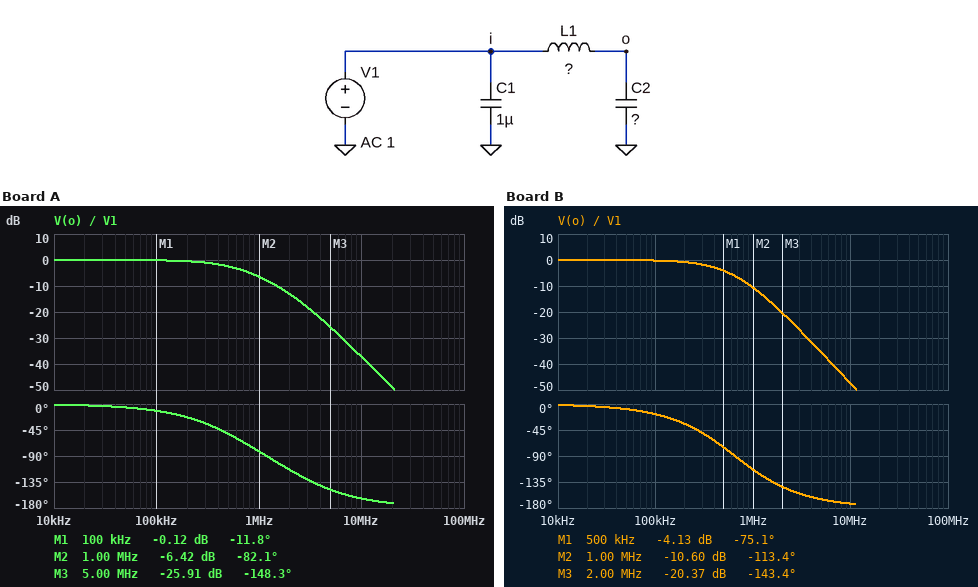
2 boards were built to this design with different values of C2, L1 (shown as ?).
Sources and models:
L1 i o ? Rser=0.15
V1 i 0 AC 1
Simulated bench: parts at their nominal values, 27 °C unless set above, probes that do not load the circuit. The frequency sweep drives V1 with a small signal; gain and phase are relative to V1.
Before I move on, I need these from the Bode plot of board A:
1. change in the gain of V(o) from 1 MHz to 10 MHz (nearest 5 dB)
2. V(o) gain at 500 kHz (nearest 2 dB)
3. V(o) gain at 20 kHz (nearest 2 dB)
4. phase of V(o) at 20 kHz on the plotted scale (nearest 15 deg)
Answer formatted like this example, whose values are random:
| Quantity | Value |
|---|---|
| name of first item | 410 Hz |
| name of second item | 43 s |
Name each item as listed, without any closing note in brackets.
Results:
| Quantity | Value |
|---|---|
| change in the gain of V(o) from 1 MHz to 10 MHz | -30 dB |
| V(o) gain at 500 kHz | -2 dB |
| V(o) gain at 20 kHz | 0 dB |
| phase of V(o) at 20 kHz on the plotted scale | 0 deg |
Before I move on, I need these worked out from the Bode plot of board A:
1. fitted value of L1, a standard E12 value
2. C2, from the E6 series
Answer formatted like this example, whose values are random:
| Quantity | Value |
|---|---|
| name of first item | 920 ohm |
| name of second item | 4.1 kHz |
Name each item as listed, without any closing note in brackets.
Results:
| Quantity | Value |
|---|---|
| fitted value of L1, a standard E12 value | 8.2 nH |
| C2, from the E6 series | 2.2 µF |
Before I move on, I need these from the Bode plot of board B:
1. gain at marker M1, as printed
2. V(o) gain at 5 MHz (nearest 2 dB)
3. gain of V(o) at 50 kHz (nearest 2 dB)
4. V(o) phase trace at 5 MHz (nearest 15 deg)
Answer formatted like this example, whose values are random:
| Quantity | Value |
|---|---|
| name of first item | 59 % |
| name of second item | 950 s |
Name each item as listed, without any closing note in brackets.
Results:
| Quantity | Value |
|---|---|
| gain at marker M1, as printed | -4.13 dB |
| V(o) gain at 5 MHz | -36 dB |
| gain of V(o) at 50 kHz | 0 dB |
| V(o) phase trace at 5 MHz | -165 deg |
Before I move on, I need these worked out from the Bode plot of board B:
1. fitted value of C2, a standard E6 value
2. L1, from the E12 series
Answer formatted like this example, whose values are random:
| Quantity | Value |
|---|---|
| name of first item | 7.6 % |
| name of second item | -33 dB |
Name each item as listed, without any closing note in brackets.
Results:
| Quantity | Value |
|---|---|
| fitted value of C2, a standard E6 value | 3.3 µF |
| L1, from the E12 series | 18 nH |
